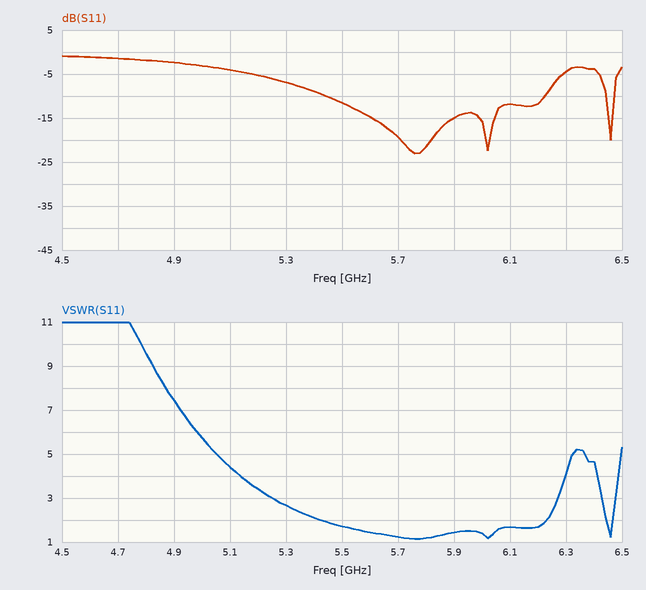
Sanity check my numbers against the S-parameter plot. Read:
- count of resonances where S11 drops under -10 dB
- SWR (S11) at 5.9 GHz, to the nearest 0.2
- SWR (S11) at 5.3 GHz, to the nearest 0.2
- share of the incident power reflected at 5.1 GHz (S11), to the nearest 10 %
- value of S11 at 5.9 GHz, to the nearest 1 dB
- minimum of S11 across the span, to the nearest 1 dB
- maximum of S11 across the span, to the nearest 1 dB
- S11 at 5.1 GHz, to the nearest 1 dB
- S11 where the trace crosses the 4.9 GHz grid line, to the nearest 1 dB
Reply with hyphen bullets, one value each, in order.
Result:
- 3
- 1.4
- 2.6
- 40 %
- -15 dB
- -23 dB
- -1 dB
- -4 dB
- -2 dB
